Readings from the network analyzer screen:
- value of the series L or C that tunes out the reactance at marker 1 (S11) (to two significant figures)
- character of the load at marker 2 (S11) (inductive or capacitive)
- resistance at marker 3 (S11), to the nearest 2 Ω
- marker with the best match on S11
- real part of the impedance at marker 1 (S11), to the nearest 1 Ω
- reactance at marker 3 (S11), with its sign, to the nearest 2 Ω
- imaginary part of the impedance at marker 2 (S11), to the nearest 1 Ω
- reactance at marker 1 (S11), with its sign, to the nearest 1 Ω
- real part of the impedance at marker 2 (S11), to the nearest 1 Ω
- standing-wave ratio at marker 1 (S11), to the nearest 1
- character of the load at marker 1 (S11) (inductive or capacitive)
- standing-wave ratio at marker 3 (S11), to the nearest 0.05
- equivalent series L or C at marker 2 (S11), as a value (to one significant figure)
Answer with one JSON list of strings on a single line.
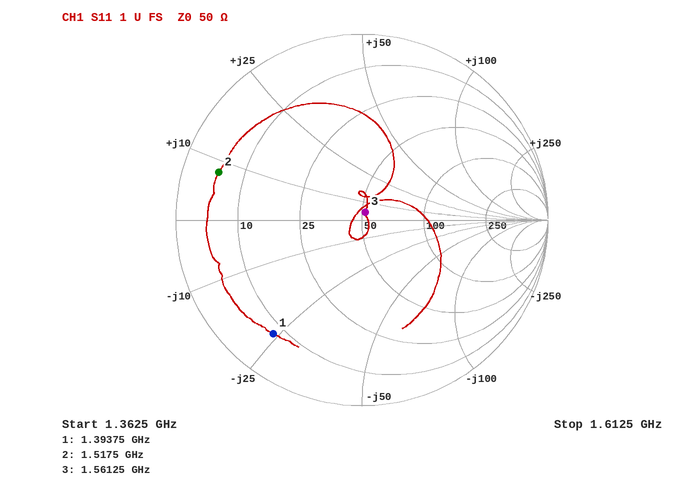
["2.7 nH", "inductive", "52 Ω", "marker 3", "8 Ω", "+4 Ω", "+8 Ω", "-24 Ω", "5 Ω", "8", "capacitive", "1.10", "800 pH"]
